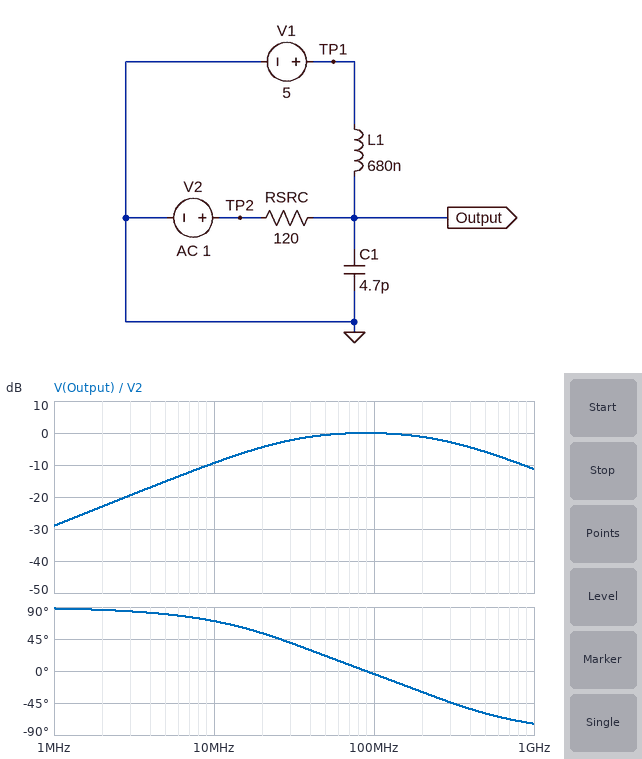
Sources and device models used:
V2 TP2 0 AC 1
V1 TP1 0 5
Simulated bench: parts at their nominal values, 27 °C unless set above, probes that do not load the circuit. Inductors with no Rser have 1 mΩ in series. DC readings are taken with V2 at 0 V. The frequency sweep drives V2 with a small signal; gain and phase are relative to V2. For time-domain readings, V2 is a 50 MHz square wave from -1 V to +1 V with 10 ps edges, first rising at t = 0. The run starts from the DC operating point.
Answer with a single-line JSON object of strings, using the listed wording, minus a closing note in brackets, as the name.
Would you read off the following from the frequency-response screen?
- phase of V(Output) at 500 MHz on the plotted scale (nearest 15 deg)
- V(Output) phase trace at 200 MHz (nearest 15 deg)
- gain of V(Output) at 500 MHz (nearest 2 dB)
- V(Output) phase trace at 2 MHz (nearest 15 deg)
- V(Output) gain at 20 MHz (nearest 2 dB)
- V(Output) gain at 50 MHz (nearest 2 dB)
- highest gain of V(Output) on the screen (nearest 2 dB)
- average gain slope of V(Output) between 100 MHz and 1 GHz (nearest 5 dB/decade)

{"phase of V(Output) at 500 MHz on the plotted scale": "-60 deg", "V(Output) phase trace at 200 MHz": "-30 deg", "gain of V(Output) at 500 MHz": "-6 dB", "V(Output) phase trace at 2 MHz": "90 deg", "V(Output) gain at 20 MHz": "-4 dB", "V(Output) gain at 50 MHz": "0 dB", "highest gain of V(Output) on the screen": "0 dB", "average gain slope of V(Output) between 100 MHz and 1 GHz": "-10 dB/decade"}
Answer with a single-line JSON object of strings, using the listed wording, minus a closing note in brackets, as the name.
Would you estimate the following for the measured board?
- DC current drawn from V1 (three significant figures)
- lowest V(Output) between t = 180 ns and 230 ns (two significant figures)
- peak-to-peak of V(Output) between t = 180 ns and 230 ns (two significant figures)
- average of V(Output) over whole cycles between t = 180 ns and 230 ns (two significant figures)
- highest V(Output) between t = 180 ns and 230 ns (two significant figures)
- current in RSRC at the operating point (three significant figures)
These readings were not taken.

{"DC current drawn from V1": "41.7 mA", "lowest V(Output) between t = 180 ns and 230 ns": "3.6 V", "peak-to-peak of V(Output) between t = 180 ns and 230 ns": "2.9 V", "average of V(Output) over whole cycles between t = 180 ns and 230 ns": "5.0 V", "highest V(Output) between t = 180 ns and 230 ns": "6.4 V", "current in RSRC at the operating point": "41.7 mA"}
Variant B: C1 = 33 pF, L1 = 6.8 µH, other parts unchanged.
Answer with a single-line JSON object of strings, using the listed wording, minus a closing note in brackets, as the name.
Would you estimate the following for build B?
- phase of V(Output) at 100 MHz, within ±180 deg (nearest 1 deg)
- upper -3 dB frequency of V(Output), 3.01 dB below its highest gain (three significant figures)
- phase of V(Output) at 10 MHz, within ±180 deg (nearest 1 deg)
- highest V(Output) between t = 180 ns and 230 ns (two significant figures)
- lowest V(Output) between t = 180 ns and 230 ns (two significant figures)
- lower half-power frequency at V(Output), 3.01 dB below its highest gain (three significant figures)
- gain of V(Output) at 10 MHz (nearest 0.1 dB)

{"phase of V(Output) at 100 MHz, within ±180 deg": "-68 deg", "upper -3 dB frequency of V(Output), 3.01 dB below its highest gain": "42.8 MHz", "phase of V(Output) at 10 MHz, within ±180 deg": "2 deg", "highest V(Output) between t = 180 ns and 230 ns": "5.9 V", "lowest V(Output) between t = 180 ns and 230 ns": "4.2 V", "lower half-power frequency at V(Output), 3.01 dB below its highest gain": "2.64 MHz", "gain of V(Output) at 10 MHz": "0 dB"}
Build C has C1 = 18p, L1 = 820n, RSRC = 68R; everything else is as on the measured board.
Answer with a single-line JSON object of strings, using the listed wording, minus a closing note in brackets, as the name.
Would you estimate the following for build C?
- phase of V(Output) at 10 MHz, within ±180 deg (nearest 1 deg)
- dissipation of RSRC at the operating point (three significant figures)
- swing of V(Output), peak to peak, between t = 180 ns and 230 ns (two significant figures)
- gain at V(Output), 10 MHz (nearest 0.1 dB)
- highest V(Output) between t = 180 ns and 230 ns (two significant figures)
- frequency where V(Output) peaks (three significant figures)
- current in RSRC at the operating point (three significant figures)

{"phase of V(Output) at 10 MHz, within ±180 deg": "51 deg", "dissipation of RSRC at the operating point": "368 mW", "swing of V(Output), peak to peak, between t = 180 ns and 230 ns": "2.3 V", "gain at V(Output), 10 MHz": "-4.1 dB", "highest V(Output) between t = 180 ns and 230 ns": "6.1 V", "frequency where V(Output) peaks": "41.4 MHz", "current in RSRC at the operating point": "73.5 mA"}
